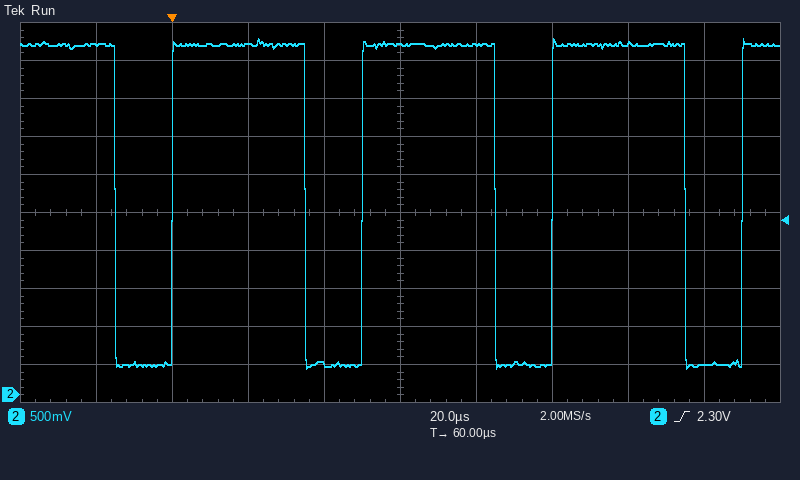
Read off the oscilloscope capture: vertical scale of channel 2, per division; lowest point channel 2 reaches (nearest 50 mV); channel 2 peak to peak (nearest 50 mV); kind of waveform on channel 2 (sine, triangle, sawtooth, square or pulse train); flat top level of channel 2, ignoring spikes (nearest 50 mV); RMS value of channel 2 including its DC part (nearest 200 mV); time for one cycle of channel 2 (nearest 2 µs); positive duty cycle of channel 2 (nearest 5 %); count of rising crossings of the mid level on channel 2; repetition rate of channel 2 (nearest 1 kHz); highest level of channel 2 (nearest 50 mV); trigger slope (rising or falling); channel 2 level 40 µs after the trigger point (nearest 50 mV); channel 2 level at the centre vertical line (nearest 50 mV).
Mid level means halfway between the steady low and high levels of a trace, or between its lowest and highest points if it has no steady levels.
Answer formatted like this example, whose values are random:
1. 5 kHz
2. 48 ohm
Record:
1. 500 mV
2. 350 mV
3. 4.35 V
4. pulse train
5. 4.60 V
6. 3.8 V
7. 50 µs
8. 70 %
9. 4
10. 20 kHz
11. 4.70 V
12. rising
13. 400 mV
14. 4.60 V
